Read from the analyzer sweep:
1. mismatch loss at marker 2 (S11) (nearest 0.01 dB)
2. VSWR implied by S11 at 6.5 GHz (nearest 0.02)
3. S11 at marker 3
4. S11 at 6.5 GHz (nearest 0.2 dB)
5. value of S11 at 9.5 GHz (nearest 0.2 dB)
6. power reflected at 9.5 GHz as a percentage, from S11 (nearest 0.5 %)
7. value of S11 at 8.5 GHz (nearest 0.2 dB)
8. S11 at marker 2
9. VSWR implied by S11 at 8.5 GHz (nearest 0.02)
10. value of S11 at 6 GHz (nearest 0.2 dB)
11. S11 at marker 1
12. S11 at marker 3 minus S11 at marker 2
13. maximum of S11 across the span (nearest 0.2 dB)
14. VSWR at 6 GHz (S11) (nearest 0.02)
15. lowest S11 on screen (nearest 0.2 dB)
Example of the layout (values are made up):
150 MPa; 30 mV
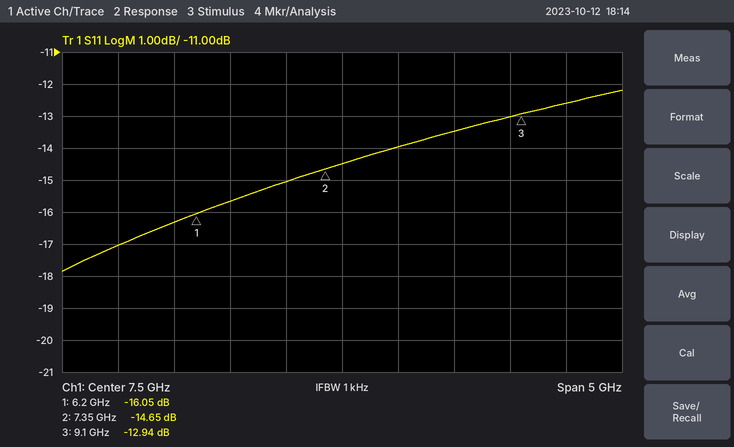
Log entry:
0.15 dB; 1.40; -12.94 dB; -15.6 dB; -12.6 dB; 5.5 %; -13.4 dB; -14.65 dB; 1.54; -16.4 dB; -16.05 dB; 1.71 dB; -12.2 dB; 1.36; -17.8 dB
